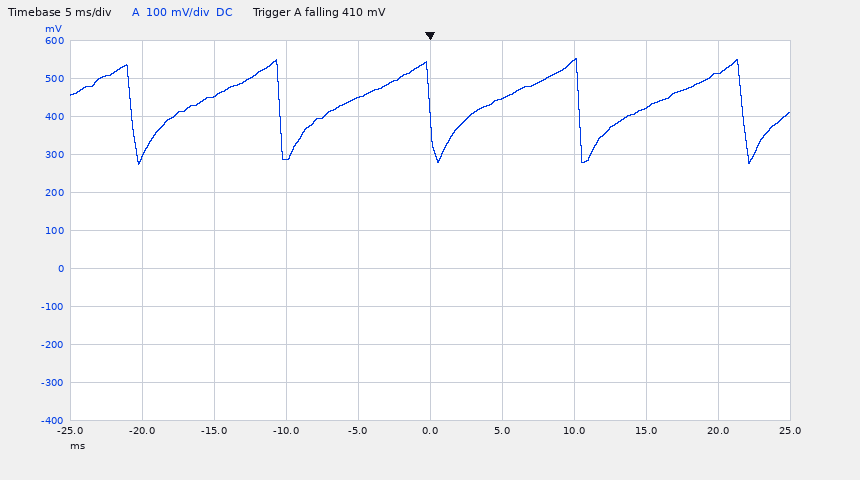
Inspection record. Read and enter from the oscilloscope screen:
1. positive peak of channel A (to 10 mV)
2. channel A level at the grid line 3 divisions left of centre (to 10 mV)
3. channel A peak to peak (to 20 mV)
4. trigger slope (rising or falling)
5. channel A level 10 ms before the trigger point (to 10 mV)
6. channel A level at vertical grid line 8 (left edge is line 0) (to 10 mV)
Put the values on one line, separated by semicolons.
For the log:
550 mV; 450 mV; 280 mV; falling; 290 mV; 420 mV
